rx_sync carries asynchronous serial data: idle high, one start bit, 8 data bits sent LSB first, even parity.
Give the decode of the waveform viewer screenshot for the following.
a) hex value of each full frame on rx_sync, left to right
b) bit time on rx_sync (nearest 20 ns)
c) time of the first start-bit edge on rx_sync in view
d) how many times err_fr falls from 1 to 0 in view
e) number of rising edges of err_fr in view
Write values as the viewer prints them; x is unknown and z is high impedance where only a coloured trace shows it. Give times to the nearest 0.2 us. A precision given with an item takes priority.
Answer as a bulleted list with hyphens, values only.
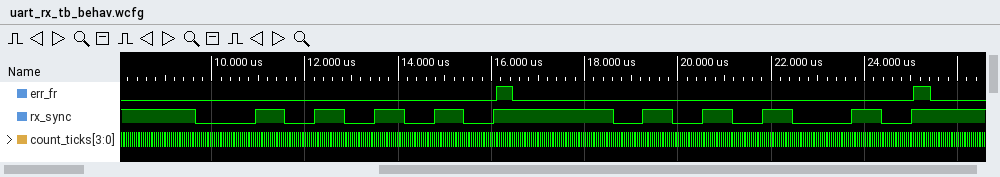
- AA, 95
- 640 ns
- 9.6 us
- 2
- 2
